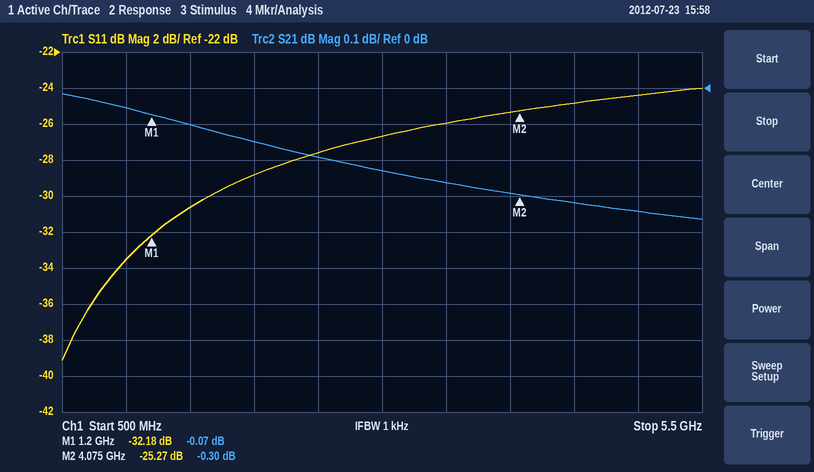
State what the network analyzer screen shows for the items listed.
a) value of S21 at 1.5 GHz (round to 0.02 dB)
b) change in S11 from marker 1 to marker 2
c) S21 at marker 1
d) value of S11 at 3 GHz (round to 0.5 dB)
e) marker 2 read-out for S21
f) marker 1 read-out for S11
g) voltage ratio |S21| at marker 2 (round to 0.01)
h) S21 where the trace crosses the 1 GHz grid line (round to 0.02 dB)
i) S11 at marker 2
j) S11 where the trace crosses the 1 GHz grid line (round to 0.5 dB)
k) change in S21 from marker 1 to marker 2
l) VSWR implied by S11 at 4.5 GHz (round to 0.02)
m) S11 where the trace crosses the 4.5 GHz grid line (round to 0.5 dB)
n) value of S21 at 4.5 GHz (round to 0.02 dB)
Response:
-0.10 dB
6.91 dB
-0.07 dB
-26.5 dB
-0.30 dB
-32.18 dB
0.97
-0.06 dB
-25.27 dB
-33.5 dB
-0.23 dB
1.12
-25.0 dB
-0.32 dB
